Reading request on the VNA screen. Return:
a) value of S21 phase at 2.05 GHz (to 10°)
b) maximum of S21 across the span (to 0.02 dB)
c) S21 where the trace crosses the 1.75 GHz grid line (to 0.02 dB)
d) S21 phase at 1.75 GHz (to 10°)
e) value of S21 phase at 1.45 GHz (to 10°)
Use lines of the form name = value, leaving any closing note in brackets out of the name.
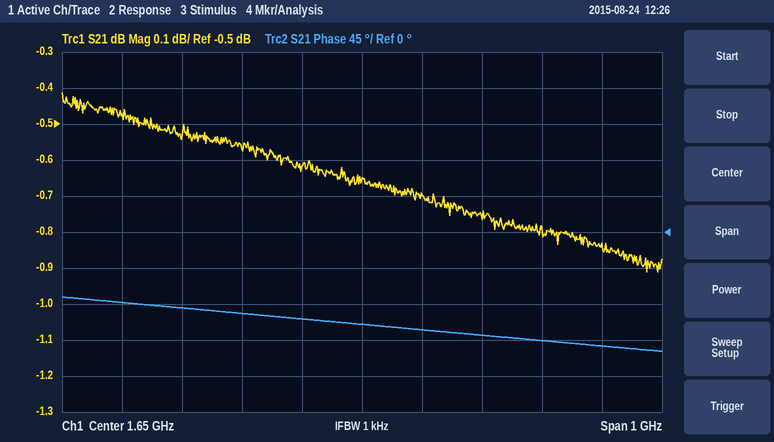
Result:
value of S21 phase at 2.05 GHz = -140°
maximum of S21 across the span = -0.42 dB
S21 where the trace crosses the 1.75 GHz grid line = -0.70 dB
S21 phase at 1.75 GHz = -120°
value of S21 phase at 1.45 GHz = -100°
